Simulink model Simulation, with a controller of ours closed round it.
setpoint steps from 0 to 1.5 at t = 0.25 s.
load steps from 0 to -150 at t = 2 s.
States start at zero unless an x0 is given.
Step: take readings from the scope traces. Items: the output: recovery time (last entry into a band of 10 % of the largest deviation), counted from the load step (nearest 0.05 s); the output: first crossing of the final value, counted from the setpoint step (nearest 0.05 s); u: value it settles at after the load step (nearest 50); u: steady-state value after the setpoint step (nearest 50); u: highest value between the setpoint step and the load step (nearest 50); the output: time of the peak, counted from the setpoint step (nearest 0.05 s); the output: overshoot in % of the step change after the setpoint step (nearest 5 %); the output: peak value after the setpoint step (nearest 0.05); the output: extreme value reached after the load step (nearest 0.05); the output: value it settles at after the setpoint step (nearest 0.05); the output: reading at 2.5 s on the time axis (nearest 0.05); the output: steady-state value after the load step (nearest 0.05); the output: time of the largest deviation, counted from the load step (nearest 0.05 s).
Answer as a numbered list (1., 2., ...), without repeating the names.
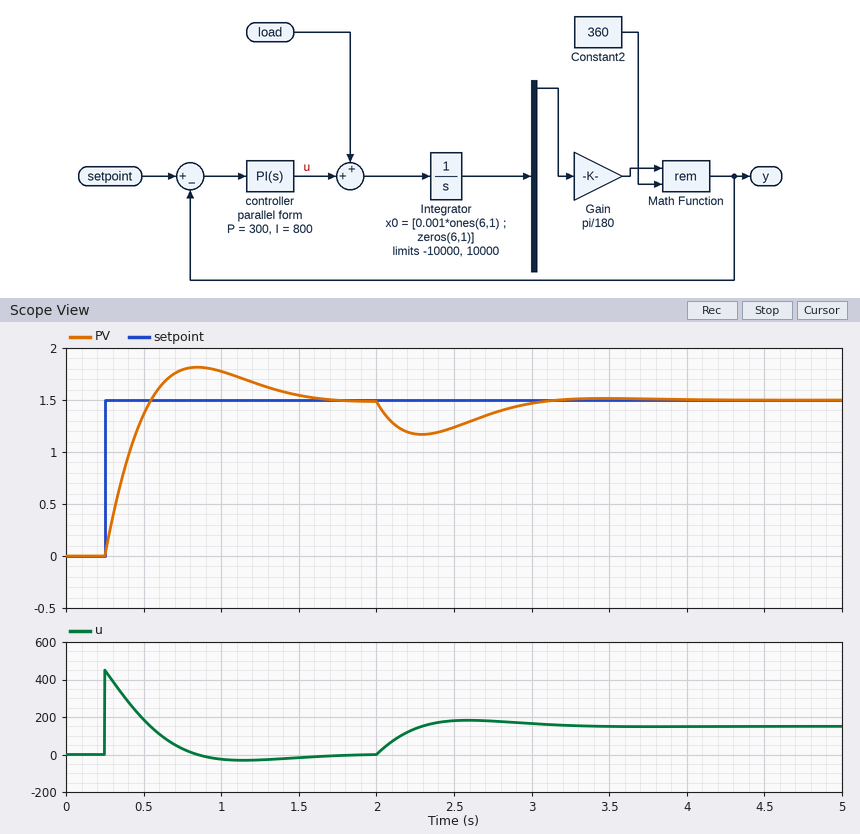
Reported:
1. 1.00 s
2. 0.30 s
3. 150
4. 0
5. 450
6. 0.60 s
7. 20 %
8. 1.80
9. 1.15
10. 1.50
11. 1.25
12. 1.50
13. 0.30 s
